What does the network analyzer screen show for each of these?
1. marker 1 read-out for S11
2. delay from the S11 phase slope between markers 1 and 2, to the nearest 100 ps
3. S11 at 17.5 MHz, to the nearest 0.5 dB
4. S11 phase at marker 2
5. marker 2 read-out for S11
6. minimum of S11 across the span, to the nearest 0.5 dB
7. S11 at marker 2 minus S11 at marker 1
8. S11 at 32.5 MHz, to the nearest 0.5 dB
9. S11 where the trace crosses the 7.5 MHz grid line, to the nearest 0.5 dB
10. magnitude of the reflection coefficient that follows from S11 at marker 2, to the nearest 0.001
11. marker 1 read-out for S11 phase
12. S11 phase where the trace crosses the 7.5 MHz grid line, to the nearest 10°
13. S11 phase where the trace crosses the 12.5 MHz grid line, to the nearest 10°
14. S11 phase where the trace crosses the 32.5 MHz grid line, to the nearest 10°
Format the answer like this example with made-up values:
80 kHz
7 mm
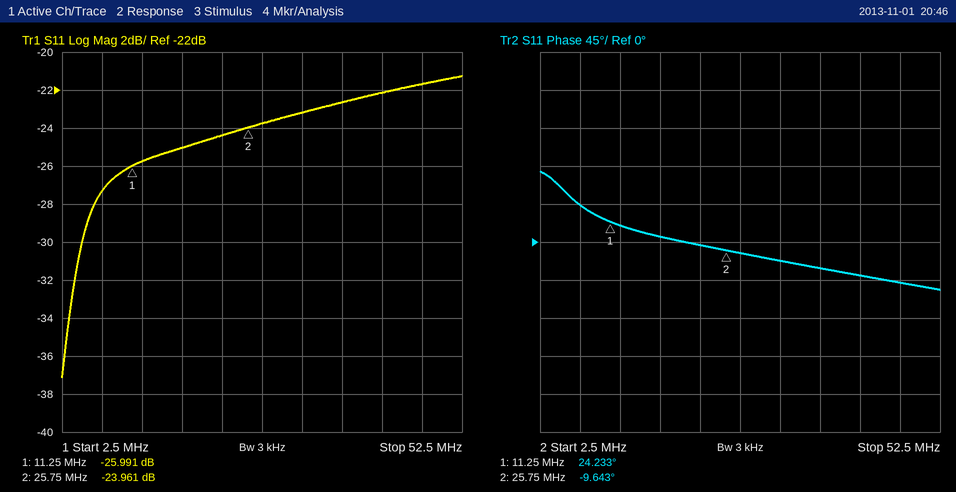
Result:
-25.991 dB
6.5 ns
-25.0 dB
-9.643°
-23.961 dB
-37.0 dB
2.030 dB
-23.0 dB
-27.5 dB
0.063
24.233°
40°
20°
-20°
